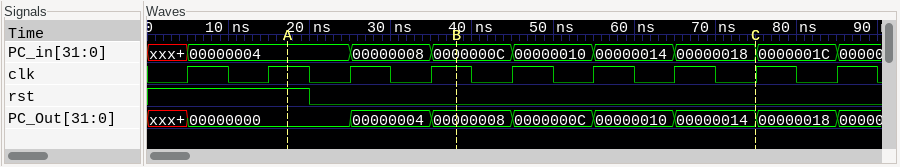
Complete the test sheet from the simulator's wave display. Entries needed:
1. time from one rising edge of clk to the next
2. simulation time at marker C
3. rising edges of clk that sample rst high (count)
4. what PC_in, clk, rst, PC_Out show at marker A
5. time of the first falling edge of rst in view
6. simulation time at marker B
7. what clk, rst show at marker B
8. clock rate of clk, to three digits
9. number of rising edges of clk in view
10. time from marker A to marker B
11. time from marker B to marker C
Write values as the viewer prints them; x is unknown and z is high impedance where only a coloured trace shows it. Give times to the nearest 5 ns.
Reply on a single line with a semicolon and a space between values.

10 ns; 75 ns; 2; PC_in=00000004, clk=1, rst=1, PC_Out=00000000; 20 ns; 40 ns; clk=1, rst=0; 100 MHz; 9; 20 ns; 35 ns
